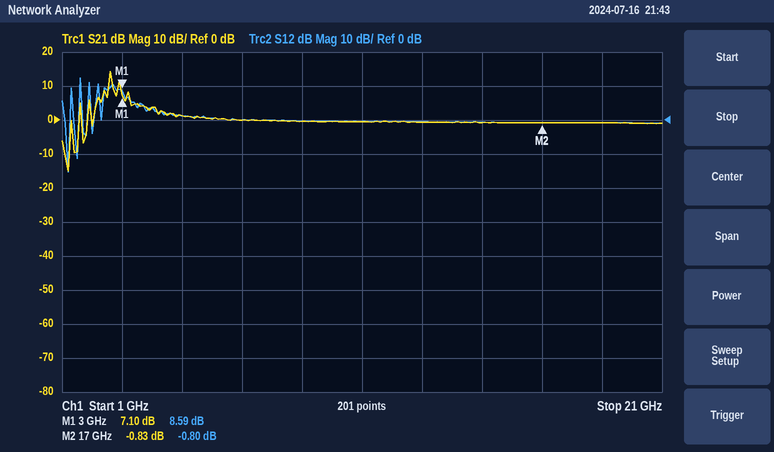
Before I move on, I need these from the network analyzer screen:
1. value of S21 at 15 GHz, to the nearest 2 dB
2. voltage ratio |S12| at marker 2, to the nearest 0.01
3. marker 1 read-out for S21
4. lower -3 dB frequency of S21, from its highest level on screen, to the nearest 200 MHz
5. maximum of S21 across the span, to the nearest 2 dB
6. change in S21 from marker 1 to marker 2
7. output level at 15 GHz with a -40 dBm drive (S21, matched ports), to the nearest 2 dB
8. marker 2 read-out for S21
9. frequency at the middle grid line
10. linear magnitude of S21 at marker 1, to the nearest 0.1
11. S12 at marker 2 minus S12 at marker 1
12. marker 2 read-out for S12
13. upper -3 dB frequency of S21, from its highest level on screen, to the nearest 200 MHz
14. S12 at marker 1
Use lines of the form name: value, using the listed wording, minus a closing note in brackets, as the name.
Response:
value of S21 at 15 GHz, to the nearest 2 dB: 0 dB
voltage ratio |S12| at marker 2, to the nearest 0.01: 0.91
marker 1 read-out for S21: 7.10 dB
lower -3 dB frequency of S21, from its highest level on screen, to the nearest 200 MHz: 2.6 GHz
maximum of S21 across the span, to the nearest 2 dB: 14 dB
change in S21 from marker 1 to marker 2: -7.93 dB
output level at 15 GHz with a -40 dBm drive (S21, matched ports), to the nearest 2 dB: -40 dBm
marker 2 read-out for S21: -0.83 dB
frequency at the middle grid line: 11 GHz
linear magnitude of S21 at marker 1, to the nearest 0.1: 2.3
S12 at marker 2 minus S12 at marker 1: -9.39 dB
marker 2 read-out for S12: -0.80 dB
upper -3 dB frequency of S21, from its highest level on screen, to the nearest 200 MHz: 2.6 GHz
S12 at marker 1: 8.59 dB
